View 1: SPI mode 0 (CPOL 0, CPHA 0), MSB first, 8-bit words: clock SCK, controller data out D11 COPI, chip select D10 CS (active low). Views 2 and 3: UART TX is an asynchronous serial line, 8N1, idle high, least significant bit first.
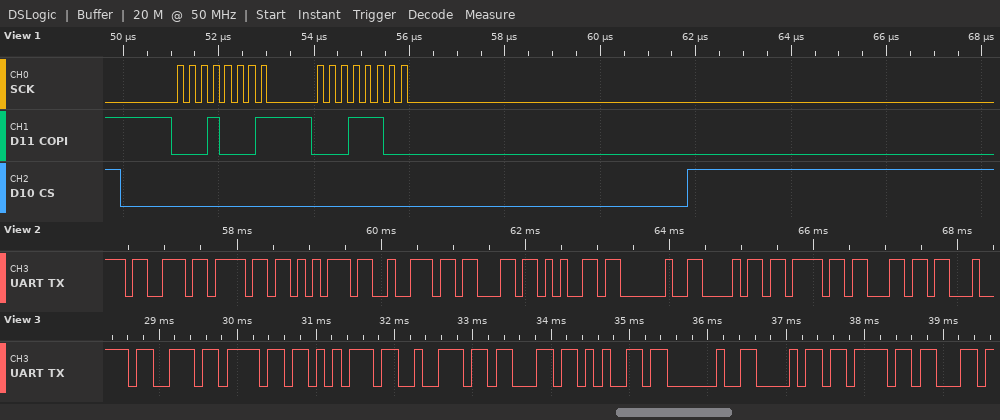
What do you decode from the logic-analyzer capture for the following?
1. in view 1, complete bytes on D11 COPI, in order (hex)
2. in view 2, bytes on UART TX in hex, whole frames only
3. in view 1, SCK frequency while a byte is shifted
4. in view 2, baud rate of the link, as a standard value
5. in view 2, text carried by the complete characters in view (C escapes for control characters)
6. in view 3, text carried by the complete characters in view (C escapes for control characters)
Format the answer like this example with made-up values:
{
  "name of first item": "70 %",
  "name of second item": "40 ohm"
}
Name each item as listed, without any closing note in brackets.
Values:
{
  "in view 1, complete bytes on D11 COPI, in order": "11 1C",
  "in view 2, bytes on UART TX in hex, whole frames only": "73 6F 75 72 63 65 20 68 6F 6C",
  "in view 1, SCK frequency while a byte is shifted": "4 MHz",
  "in view 2, baud rate of the link, as a standard value": "9600 baud",
  "in view 2, text carried by the complete characters in view": "\"source hol\"",
  "in view 3, text carried by the complete characters in view": "\"source ho\""
}
